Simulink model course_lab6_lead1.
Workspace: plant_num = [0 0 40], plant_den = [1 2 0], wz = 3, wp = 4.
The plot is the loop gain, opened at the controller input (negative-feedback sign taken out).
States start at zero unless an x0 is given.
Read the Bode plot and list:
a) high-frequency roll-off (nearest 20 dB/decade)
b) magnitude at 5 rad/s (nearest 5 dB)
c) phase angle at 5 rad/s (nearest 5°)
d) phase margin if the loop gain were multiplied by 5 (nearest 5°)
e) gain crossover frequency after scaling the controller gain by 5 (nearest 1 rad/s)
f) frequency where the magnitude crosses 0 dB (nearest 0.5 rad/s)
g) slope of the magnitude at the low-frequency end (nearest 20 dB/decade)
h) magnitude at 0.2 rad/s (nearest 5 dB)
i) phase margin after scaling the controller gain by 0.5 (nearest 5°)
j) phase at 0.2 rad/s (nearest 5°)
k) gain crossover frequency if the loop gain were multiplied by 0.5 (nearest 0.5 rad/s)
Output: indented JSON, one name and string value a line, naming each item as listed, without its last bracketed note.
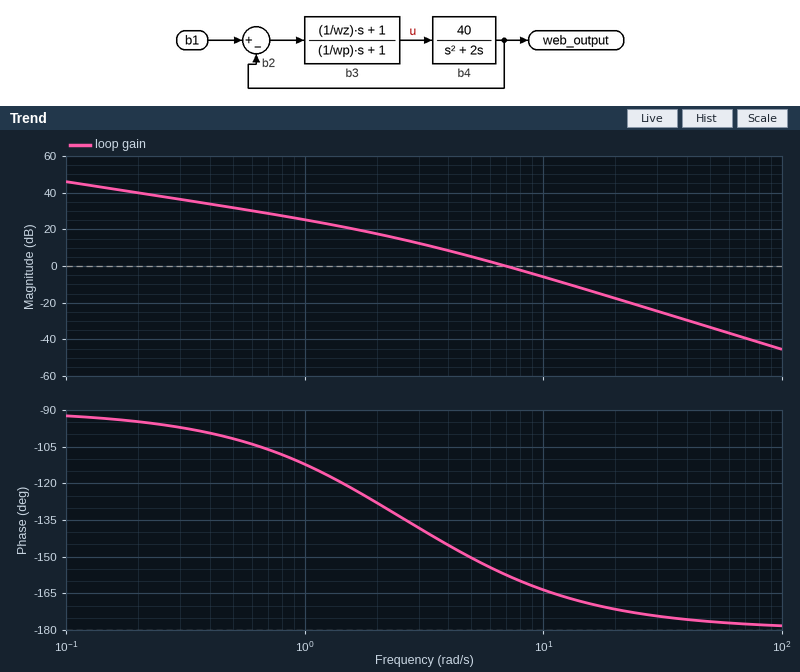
{
  "high-frequency roll-off": "-40 dB/decade",
  "magnitude at 5 rad/s": "5 dB",
  "phase angle at 5 rad/s": "-150°",
  "phase margin if the loop gain were multiplied by 5": "10°",
  "gain crossover frequency after scaling the controller gain by 5": "16 rad/s",
  "frequency where the magnitude crosses 0 dB": "7.0 rad/s",
  "slope of the magnitude at the low-frequency end": "-20 dB/decade",
  "magnitude at 0.2 rad/s": "40 dB",
  "phase margin after scaling the controller gain by 0.5": "30°",
  "phase at 0.2 rad/s": "-95°",
  "gain crossover frequency if the loop gain were multiplied by 0.5": "4.5 rad/s"
}
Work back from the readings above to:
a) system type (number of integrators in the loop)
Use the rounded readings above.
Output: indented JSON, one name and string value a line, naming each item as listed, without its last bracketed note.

{
  "system type": "1"
}
